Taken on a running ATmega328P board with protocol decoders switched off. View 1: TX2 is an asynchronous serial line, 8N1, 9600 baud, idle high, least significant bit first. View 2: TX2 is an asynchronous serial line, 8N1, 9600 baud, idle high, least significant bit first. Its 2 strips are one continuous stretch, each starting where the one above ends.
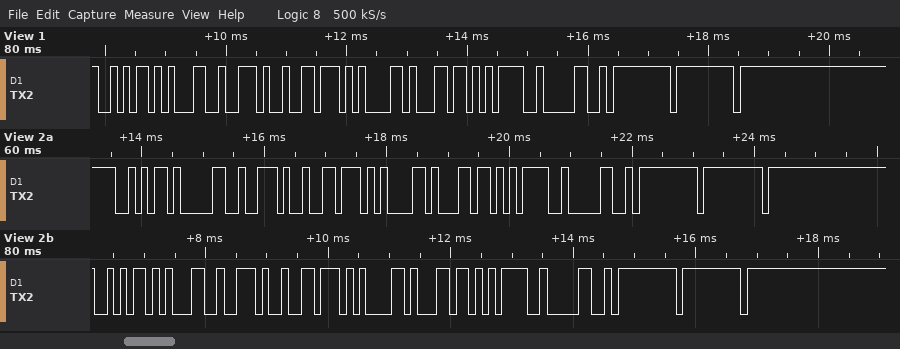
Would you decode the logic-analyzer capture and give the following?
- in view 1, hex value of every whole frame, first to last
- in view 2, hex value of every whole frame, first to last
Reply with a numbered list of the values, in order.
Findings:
1. 6A 31 2E 76 61 6C 3D 30 FF FF FF
2. 6A 30 2E 76 61 6C 3D 30 FF FF FF 6A 31 2E 76 61 6C 3D 30 FF FF FF
